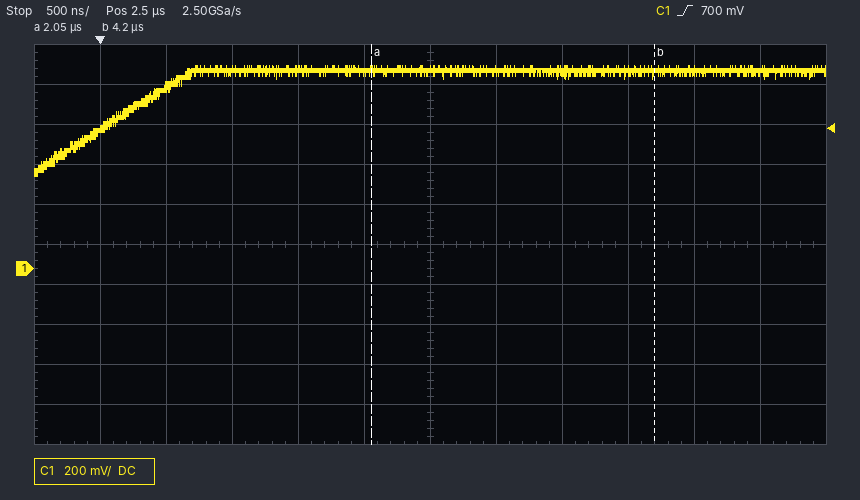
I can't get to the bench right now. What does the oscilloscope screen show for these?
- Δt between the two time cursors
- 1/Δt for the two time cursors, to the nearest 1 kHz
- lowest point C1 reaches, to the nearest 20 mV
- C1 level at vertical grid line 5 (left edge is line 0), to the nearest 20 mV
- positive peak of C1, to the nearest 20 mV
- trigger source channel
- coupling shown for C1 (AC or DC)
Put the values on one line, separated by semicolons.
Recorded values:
2.15 µs; 465 kHz; 460 mV; 980 mV; 1.02 V; C1; DC
